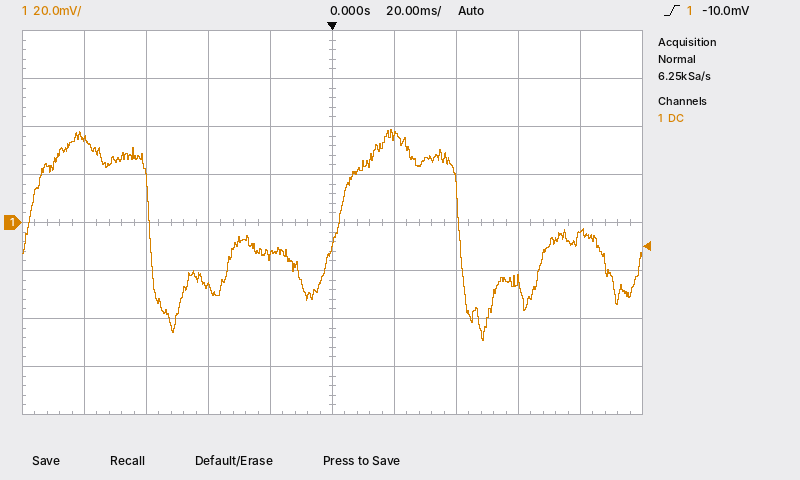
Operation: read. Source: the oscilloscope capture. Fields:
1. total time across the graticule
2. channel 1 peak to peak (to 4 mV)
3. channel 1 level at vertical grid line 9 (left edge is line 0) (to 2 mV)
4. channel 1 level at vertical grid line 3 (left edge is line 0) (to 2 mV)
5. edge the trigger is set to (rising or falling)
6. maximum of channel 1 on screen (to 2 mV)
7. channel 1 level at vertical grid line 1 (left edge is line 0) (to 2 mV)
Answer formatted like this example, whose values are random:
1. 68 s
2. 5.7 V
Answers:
1. 200 ms
2. 88 mV
3. -4 mV
4. -26 mV
5. rising
6. 38 mV
7. 34 mV
